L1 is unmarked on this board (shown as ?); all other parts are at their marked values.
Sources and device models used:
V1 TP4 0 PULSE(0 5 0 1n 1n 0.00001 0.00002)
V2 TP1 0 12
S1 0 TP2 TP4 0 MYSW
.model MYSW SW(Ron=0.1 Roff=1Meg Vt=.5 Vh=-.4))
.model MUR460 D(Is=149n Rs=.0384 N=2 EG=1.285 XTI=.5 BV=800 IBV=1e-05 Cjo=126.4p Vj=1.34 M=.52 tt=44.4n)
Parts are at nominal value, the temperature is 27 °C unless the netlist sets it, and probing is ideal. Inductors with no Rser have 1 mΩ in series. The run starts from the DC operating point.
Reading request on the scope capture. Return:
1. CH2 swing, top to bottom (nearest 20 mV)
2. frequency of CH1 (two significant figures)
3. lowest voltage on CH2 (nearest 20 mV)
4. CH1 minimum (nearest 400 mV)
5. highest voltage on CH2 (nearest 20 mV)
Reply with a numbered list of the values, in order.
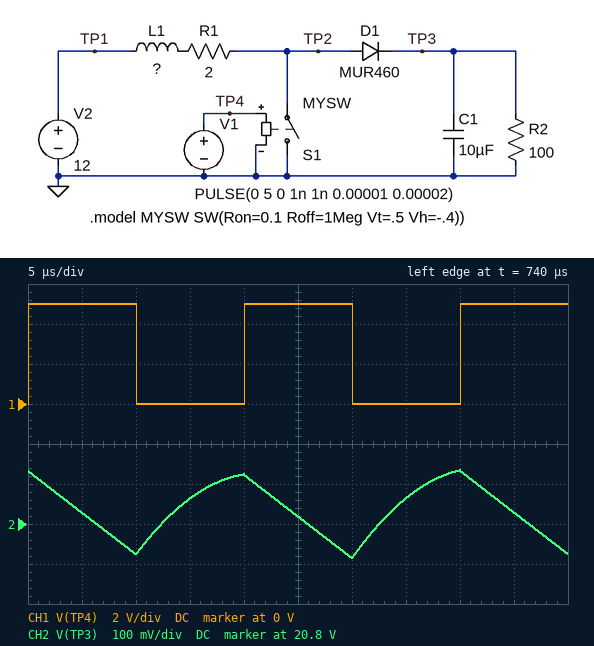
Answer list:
1. 220 mV
2. 50 kHz
3. 20.72 V
4. 0 V
5. 20.94 V
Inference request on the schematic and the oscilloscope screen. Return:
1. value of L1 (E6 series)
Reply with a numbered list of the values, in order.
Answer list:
1. 330 µH
